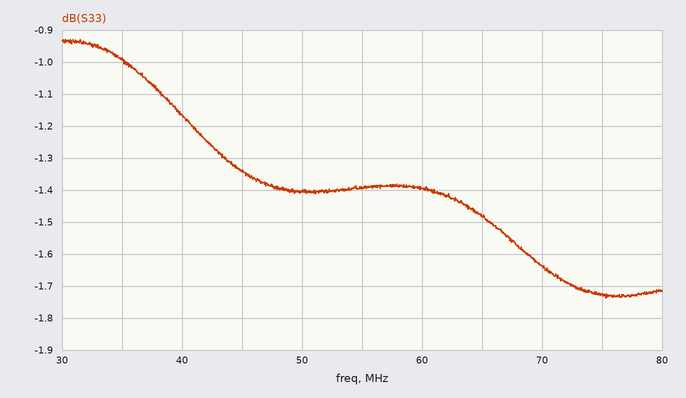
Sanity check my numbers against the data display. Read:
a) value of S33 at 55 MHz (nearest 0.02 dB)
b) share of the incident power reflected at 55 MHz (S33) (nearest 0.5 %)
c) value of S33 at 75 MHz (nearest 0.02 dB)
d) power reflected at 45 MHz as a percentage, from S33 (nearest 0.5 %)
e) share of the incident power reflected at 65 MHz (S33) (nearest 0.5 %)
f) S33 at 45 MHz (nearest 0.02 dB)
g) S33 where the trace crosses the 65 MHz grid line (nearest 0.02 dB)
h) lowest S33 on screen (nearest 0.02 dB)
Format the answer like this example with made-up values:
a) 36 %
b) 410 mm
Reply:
a) -1.40 dB
b) 72.5 %
c) -1.72 dB
d) 73.5 %
e) 71.0 %
f) -1.34 dB
g) -1.48 dB
h) -1.74 dB
